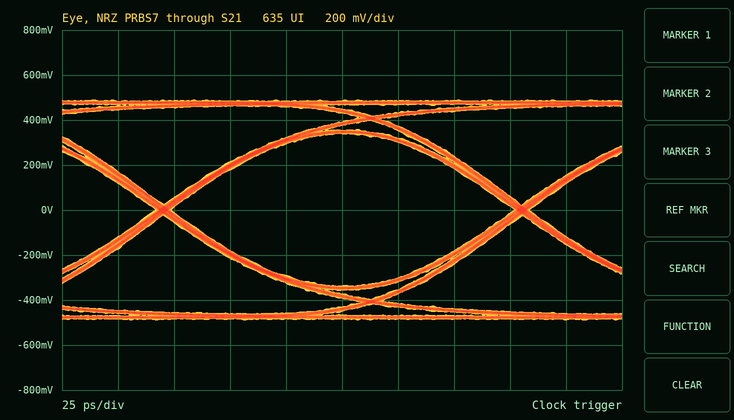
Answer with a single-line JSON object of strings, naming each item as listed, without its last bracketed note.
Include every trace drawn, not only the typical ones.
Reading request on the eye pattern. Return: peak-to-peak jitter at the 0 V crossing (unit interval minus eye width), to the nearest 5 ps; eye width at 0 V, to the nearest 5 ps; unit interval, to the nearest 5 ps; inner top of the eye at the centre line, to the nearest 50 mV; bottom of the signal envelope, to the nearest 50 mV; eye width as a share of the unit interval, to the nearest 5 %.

{"peak-to-peak jitter at the 0 V crossing (unit interval minus eye width), to the nearest 5 ps": "5 ps", "eye width at 0 V, to the nearest 5 ps": "155 ps", "unit interval, to the nearest 5 ps": "160 ps", "inner top of the eye at the centre line, to the nearest 50 mV": "350 mV", "bottom of the signal envelope, to the nearest 50 mV": "-500 mV", "eye width as a share of the unit interval, to the nearest 5 %": "95 %"}
